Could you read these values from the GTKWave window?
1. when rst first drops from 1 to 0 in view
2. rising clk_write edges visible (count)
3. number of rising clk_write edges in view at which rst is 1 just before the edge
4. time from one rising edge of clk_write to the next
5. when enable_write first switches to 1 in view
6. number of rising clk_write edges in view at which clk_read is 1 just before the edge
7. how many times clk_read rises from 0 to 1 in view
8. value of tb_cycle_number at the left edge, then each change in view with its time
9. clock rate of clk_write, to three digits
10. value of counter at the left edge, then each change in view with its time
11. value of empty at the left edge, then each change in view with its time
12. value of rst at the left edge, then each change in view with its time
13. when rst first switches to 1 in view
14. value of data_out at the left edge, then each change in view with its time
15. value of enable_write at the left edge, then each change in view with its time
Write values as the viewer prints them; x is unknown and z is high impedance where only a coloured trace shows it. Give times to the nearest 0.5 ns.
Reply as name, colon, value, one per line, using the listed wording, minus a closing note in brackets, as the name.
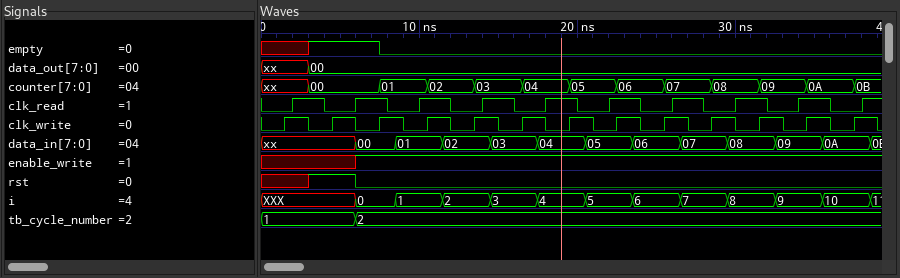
when rst first drops from 1 to 0 in view: 6 ns
rising clk_write edges visible: 13
number of rising clk_write edges in view at which rst is 1 just before the edge: 1
time from one rising edge of clk_write to the next: 3 ns
when enable_write first switches to 1 in view: 6 ns
number of rising clk_write edges in view at which clk_read is 1 just before the edge: 6
how many times clk_read rises from 0 to 1 in view: 10
value of tb_cycle_number at the left edge, then each change in view with its time: 1, 2 at 6 ns
clock rate of clk_write, to three digits: 333 MHz
value of counter at the left edge, then each change in view with its time: xx, 00 at 3 ns, 01 at 7.5 ns, 02 at 10.5 ns, 03 at 13.5 ns, 04 at 16.5 ns, 05 at 19.5 ns, 06 at 22.5 ns, 07 at 25.5 ns, 08 at 28.5 ns, 09 at 31.5 ns, 0A at 34.5 ns, 0B at 37.5 ns
value of empty at the left edge, then each change in view with its time: x, 1 at 3 ns, 0 at 7.5 ns
value of rst at the left edge, then each change in view with its time: x, 1 at 3 ns, 0 at 6 ns
when rst first switches to 1 in view: 3 ns
value of data_out at the left edge, then each change in view with its time: xx, 00 at 3 ns
value of enable_write at the left edge, then each change in view with its time: x, 1 at 6 ns
